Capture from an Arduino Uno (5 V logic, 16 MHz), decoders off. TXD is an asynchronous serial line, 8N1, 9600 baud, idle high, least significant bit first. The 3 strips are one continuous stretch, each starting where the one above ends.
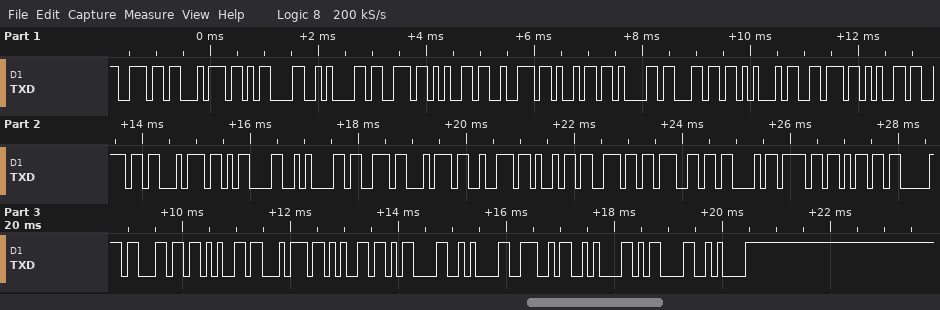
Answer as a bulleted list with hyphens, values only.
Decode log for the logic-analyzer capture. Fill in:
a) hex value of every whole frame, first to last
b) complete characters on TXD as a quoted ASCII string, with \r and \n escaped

- 0x6E 0x74 0x0D 0x0A 0x73 0x65 0x72 0x69 0x61 0x6C 0x45 0x76 0x65 0x6E 0x74 0x0D 0x0A 0x73 0x74 0x72 0x69 0x6E 0x67 0x43 0x6F 0x6D 0x70 0x6C 0x65 0x74 0x65 0x0D 0x0A 0x4E 0x0A 0x0D 0x0A
- "nt\r\nserialEvent\r\nstringComplete\r\nN\n\r\n"
